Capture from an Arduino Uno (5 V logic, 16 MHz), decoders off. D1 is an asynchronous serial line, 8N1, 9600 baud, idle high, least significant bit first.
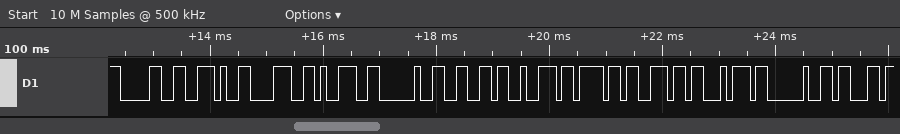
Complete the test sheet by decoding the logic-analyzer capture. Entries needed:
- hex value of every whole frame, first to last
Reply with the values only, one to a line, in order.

0x30 0x2E 0x38 0x39 0x20 0x66 0x72 0x6F 0x6E 0x74 0x20 0x63
